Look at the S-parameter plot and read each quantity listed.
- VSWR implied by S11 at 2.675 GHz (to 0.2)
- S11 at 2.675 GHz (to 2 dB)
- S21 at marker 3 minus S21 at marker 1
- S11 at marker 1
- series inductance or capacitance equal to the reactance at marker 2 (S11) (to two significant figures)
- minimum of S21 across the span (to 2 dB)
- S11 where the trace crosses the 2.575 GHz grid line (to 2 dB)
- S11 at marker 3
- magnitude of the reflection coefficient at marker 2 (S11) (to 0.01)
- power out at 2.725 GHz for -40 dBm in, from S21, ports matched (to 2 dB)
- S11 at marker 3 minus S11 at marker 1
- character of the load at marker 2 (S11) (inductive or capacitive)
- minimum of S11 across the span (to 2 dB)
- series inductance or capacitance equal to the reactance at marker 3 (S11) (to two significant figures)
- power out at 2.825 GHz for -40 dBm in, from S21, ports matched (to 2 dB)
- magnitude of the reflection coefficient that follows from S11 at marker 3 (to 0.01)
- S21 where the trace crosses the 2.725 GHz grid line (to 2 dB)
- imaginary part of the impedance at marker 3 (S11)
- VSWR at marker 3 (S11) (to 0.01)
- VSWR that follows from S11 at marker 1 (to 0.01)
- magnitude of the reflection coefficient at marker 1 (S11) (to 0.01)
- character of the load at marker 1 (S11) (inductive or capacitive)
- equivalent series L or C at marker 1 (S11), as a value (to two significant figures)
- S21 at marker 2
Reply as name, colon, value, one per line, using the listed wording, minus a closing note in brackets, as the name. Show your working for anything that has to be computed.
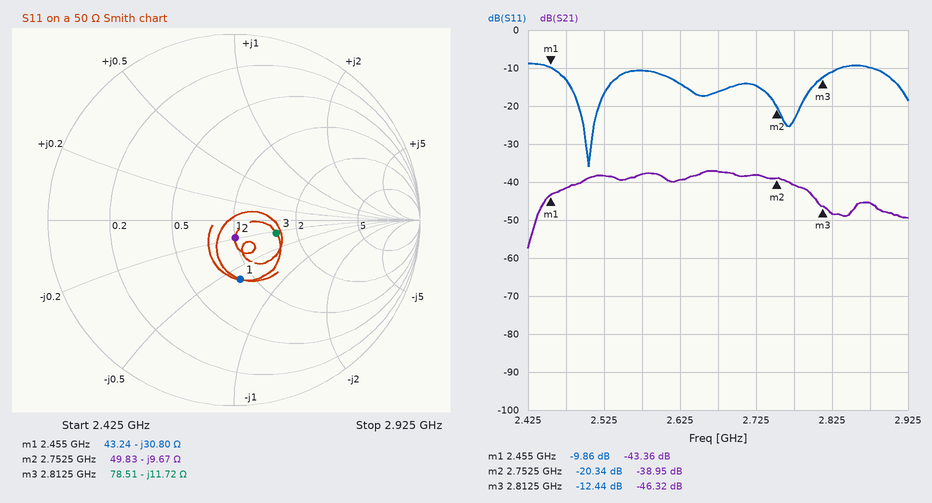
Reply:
VSWR implied by S11 at 2.675 GHz: |Γ| = 10^(-16/20) = 0.1585; VSWR = (1 + 0.1585)/(1 − 0.1585) ≈ 1.4
S11 at 2.675 GHz: -16 dB
S21 at marker 3 minus S21 at marker 1: -46.32 − (-43.36) = -2.96 dB
S11 at marker 1: -9.86 dB
series inductance or capacitance equal to the reactance at marker 2 (S11): C = 1/(2π × 2.7525 GHz × 9.67 Ω) ≈ 6.0 pF
minimum of S21 across the span: -58 dB
S11 where the trace crosses the 2.575 GHz grid line: -10 dB
S11 at marker 3: -12.44 dB
magnitude of the reflection coefficient at marker 2 (S11): 0.10
power out at 2.725 GHz for -40 dBm in, from S21, ports matched: -40 dBm + (-38 dB) = -78 dBm
S11 at marker 3 minus S11 at marker 1: -12.44 − (-9.86) = -2.58 dB
character of the load at marker 2 (S11): capacitive
minimum of S11 across the span: -36 dB
series inductance or capacitance equal to the reactance at marker 3 (S11): C = 1/(2π × 2.8125 GHz × 11.72 Ω) ≈ 4.8 pF
power out at 2.825 GHz for -40 dBm in, from S21, ports matched: -40 dBm + (-48 dB) = -88 dBm
magnitude of the reflection coefficient that follows from S11 at marker 3: 10^(-12.44/20) ≈ 0.24
S21 where the trace crosses the 2.725 GHz grid line: -38 dB
imaginary part of the impedance at marker 3: -11.72 Ω
VSWR at marker 3 (S11): 1.63
VSWR that follows from S11 at marker 1: (1 + 0.3214)/(1 − 0.3214) ≈ 1.95
magnitude of the reflection coefficient at marker 1 (S11): 0.32
character of the load at marker 1 (S11): capacitive
equivalent series L or C at marker 1 (S11), as a value: C = 1/(2π × 2.455 GHz × 30.8 Ω) ≈ 2.1 pF
S21 at marker 2: -38.95 dB
